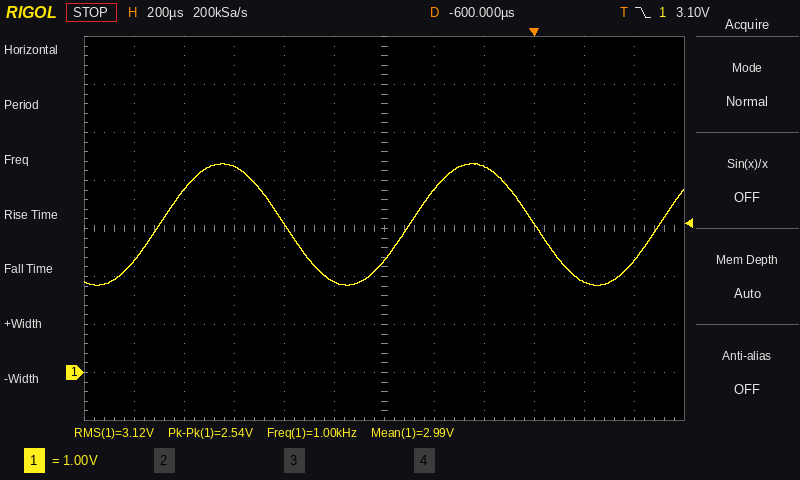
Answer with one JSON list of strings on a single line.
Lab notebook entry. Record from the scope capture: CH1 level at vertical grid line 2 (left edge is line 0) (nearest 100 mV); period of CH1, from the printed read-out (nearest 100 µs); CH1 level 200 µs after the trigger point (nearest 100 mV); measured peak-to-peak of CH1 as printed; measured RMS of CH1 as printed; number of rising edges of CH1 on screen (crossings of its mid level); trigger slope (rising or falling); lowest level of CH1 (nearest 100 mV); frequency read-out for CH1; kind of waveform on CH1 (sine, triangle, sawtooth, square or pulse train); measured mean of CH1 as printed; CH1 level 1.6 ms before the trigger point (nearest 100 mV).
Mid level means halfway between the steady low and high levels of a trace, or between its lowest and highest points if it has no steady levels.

["3.8 V", "1.0 ms", "1.9 V", "2.54 V", "3.12 V", "3", "falling", "1.8 V", "1.00 kHz", "sine", "2.99 V", "2.3 V"]
